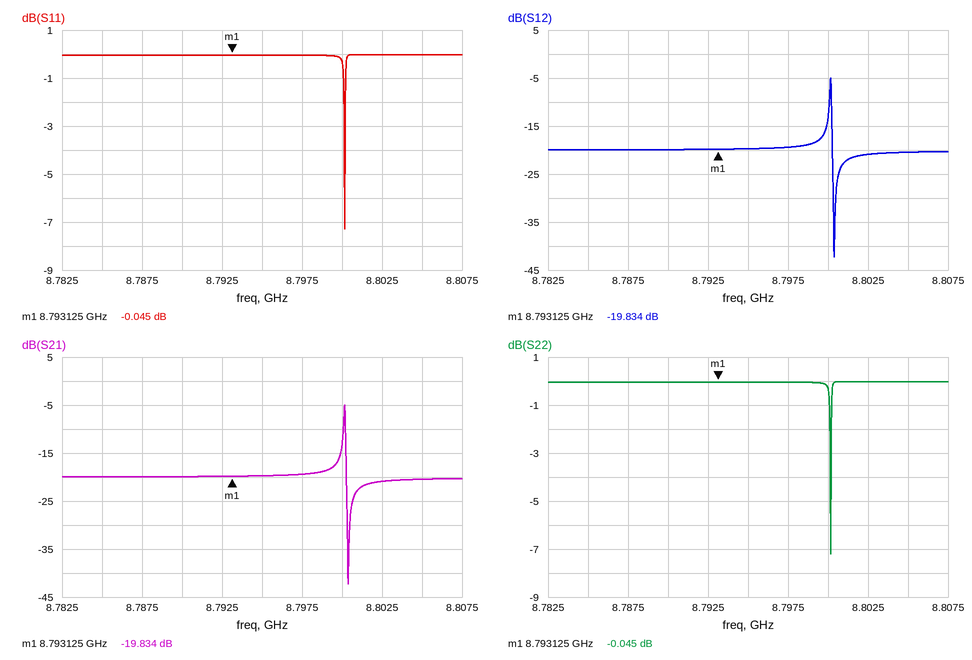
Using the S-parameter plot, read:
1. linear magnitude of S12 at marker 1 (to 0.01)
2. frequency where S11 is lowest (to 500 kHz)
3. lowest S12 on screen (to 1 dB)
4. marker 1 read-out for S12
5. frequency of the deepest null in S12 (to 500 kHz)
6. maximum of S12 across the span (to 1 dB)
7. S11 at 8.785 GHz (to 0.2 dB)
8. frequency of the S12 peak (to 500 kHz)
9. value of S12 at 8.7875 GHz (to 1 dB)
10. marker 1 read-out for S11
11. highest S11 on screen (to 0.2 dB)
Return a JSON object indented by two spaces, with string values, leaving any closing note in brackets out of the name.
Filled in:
{
  "linear magnitude of S12 at marker 1": "0.10",
  "frequency where S11 is lowest": "8.8000 GHz",
  "lowest S12 on screen": "-42 dB",
  "marker 1 read-out for S12": "-19.834 dB",
  "frequency of the deepest null in S12": "8.8005 GHz",
  "maximum of S12 across the span": "-5 dB",
  "S11 at 8.785 GHz": "0.0 dB",
  "frequency of the S12 peak": "8.8000 GHz",
  "value of S12 at 8.7875 GHz": "-20 dB",
  "marker 1 read-out for S11": "-0.045 dB",
  "highest S11 on screen": "0.0 dB"
}
